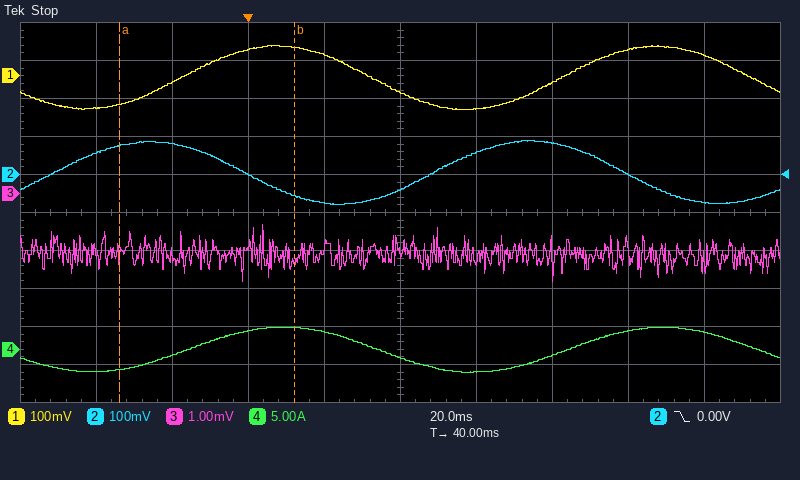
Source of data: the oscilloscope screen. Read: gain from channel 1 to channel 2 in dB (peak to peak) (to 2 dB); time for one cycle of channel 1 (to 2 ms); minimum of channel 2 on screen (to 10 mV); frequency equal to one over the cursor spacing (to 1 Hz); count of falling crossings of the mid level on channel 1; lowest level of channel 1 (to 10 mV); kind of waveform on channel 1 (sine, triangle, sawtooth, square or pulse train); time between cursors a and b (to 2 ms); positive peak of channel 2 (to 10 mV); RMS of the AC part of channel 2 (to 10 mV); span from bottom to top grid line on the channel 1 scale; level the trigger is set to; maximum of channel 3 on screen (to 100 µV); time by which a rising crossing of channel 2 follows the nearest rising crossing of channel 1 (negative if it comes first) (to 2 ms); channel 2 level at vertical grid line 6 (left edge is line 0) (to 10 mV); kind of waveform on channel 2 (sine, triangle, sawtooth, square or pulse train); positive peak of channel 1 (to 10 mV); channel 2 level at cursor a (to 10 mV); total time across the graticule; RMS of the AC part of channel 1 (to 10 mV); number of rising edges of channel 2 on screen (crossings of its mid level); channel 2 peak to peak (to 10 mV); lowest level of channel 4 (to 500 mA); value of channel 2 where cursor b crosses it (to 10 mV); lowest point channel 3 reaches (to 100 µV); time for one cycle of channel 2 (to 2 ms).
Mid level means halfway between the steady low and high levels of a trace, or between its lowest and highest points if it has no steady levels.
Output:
0 dB
100 ms
-80 mV
22 Hz
2
-90 mV
sine
46 ms
90 mV
60 mV
1 V
0.00 V
-800 µV
-34 ms
60 mV
sine
80 mV
80 mV
200 ms
60 mV
2
170 mV
-3.0 A
-60 mV
-2.3 mV
100 ms
